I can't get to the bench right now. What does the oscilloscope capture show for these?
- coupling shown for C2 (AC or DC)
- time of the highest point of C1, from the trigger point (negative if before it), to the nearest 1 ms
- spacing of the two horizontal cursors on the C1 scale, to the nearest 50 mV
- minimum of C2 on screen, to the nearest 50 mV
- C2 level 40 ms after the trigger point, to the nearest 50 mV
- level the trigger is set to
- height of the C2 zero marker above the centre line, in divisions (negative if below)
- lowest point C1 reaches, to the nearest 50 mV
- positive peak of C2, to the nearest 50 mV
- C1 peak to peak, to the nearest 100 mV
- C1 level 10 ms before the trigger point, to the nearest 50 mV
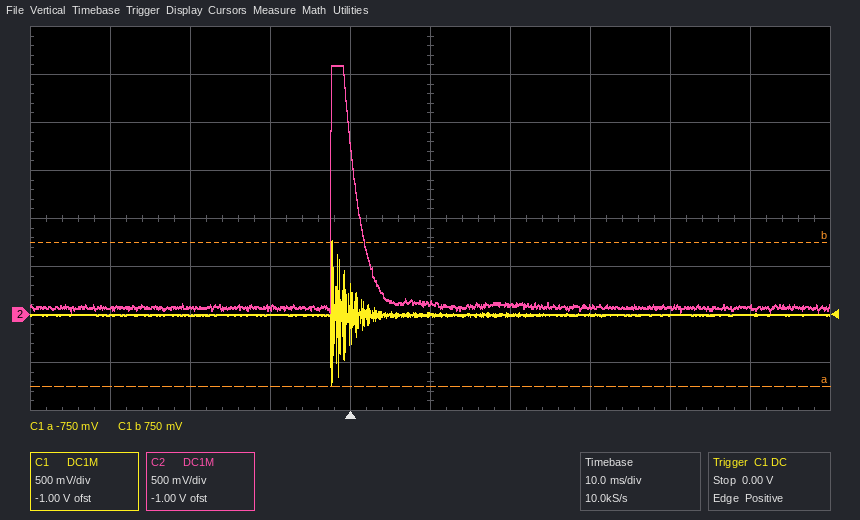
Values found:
DC
-2 ms
1.50 V
0 mV
50 mV
0.00 V
-2.0 div
-750 mV
2.60 V
1.50 V
0 mV
